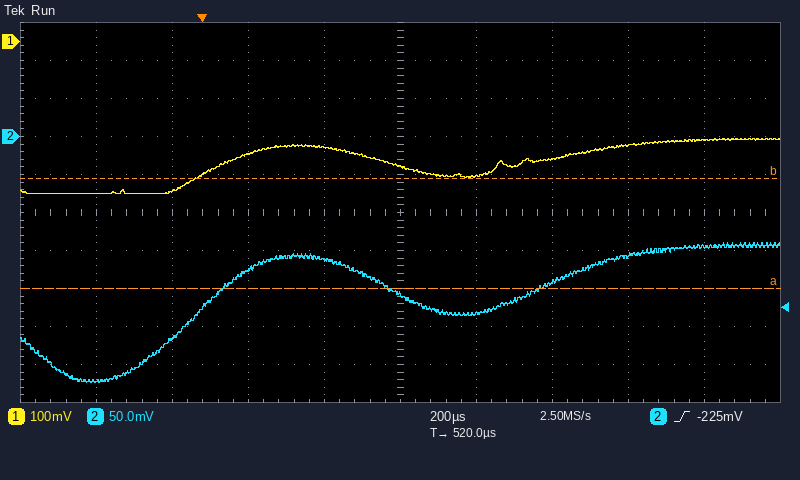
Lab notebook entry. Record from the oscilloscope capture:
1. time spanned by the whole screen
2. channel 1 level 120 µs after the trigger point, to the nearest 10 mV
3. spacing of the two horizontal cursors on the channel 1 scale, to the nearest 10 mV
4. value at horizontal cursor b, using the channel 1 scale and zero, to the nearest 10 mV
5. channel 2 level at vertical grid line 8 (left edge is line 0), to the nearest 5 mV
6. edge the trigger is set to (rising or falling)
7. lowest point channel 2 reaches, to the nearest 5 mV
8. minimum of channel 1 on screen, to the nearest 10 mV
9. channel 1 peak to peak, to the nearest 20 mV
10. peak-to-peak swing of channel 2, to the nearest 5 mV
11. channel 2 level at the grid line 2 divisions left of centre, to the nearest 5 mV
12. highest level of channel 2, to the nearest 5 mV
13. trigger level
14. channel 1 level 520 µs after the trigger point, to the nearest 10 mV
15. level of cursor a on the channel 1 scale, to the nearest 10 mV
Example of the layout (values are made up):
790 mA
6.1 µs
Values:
2 ms
-300 mV
290 mV
-360 mV
-155 mV
rising
-325 mV
-400 mV
140 mV
185 mV
-175 mV
-140 mV
-225 mV
-330 mV
-650 mV
